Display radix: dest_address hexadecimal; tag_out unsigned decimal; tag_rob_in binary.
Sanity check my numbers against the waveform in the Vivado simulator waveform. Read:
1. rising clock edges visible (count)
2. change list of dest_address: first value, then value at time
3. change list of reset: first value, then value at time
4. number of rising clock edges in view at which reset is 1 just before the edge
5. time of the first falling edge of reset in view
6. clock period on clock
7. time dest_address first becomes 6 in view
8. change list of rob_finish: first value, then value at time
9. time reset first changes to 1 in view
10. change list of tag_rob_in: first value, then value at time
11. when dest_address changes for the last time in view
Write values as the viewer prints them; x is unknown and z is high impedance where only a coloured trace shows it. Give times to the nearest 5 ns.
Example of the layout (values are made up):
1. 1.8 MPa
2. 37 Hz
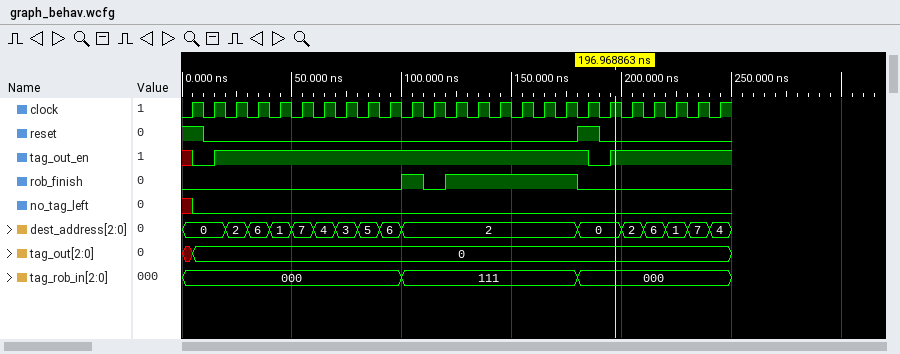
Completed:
1. 25
2. 0, 2 at 20 ns, 6 at 30 ns, 1 at 40 ns, 7 at 50 ns, 4 at 60 ns, 3 at 70 ns, 5 at 80 ns, 6 at 90 ns, 2 at 100 ns, 0 at 180 ns, 2 at 200 ns, 6 at 210 ns, 1 at 220 ns, 7 at 230 ns, 4 at 240 ns
3. 1, 0 at 10 ns, 1 at 180 ns, 0 at 190 ns
4. 2
5. 10 ns
6. 10 ns
7. 30 ns
8. 0, 1 at 100 ns, 0 at 110 ns, 1 at 120 ns, 0 at 180 ns
9. 180 ns
10. 000, 111 at 100 ns, 000 at 180 ns
11. 240 ns
